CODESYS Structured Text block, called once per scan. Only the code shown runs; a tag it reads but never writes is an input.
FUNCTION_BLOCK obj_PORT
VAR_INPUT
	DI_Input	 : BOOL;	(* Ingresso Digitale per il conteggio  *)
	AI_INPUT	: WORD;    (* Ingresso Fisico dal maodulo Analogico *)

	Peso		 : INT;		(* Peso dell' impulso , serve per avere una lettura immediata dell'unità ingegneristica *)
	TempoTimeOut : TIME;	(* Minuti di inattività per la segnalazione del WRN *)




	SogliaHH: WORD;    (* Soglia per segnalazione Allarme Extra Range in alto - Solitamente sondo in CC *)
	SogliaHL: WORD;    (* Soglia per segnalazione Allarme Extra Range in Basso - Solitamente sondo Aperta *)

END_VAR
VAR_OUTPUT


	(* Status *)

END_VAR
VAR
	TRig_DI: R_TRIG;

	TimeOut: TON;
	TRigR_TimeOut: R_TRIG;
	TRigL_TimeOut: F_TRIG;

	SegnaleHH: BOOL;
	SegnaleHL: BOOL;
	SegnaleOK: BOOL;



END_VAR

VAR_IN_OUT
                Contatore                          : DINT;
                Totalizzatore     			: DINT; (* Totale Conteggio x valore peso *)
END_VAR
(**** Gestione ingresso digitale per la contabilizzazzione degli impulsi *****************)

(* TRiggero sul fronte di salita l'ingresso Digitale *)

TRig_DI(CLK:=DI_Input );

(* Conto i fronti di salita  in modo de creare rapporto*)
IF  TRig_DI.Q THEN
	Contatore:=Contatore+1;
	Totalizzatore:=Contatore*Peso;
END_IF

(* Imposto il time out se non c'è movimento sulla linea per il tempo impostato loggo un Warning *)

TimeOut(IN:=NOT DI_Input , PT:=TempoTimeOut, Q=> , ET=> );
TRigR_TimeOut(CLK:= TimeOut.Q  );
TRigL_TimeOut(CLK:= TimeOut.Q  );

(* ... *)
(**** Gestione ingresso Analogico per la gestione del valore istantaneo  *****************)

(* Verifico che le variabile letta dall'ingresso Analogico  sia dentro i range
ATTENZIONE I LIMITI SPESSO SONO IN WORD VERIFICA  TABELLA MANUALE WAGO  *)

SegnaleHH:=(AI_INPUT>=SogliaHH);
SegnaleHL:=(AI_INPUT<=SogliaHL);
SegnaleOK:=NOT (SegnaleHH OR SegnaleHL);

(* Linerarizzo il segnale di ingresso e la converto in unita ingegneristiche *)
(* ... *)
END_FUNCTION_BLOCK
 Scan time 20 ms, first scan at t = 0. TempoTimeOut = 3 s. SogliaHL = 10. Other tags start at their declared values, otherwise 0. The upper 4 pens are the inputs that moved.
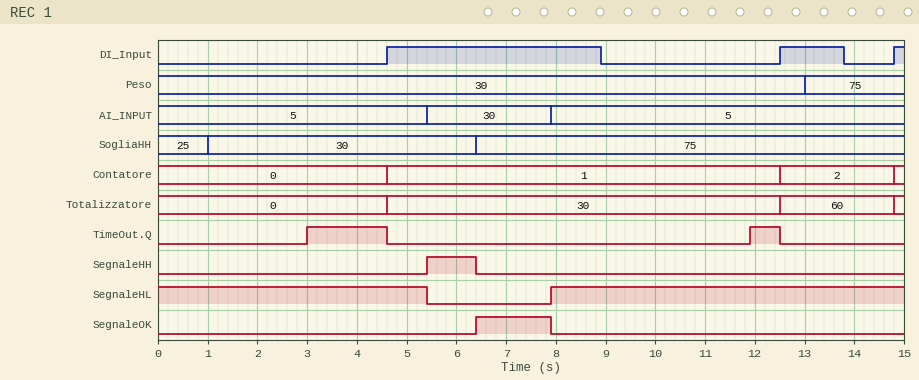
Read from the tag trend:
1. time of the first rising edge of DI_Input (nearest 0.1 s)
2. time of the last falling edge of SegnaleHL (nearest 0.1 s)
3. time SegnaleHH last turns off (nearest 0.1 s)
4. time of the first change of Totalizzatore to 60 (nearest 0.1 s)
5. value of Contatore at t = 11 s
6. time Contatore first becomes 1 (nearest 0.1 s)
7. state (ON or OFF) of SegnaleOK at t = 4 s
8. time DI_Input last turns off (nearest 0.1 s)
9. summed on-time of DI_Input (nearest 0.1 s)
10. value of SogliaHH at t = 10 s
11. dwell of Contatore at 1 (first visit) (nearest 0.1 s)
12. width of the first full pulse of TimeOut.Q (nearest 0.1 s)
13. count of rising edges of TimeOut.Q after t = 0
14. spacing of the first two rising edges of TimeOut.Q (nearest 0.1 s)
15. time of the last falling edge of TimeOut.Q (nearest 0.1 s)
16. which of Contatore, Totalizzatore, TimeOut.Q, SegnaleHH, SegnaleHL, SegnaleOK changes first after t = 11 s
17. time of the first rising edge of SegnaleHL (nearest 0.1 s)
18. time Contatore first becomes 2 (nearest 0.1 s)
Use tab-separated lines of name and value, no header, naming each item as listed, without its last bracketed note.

time of the first rising edge of DI_Input	4.6 s
time of the last falling edge of SegnaleHL	5.4 s
time SegnaleHH last turns off	6.4 s
time of the first change of Totalizzatore to 60	12.5 s
value of Contatore at t = 11 s	1
time Contatore first becomes 1	4.6 s
state (ON or OFF) of SegnaleOK at t = 4 s	OFF
time DI_Input last turns off	13.8 s
summed on-time of DI_Input	5.8 s
value of SogliaHH at t = 10 s	75
dwell of Contatore at 1 (first visit)	7.9 s
width of the first full pulse of TimeOut.Q	1.6 s
count of rising edges of TimeOut.Q after t = 0	2
spacing of the first two rising edges of TimeOut.Q	8.9 s
time of the last falling edge of TimeOut.Q	12.5 s
which of Contatore, Totalizzatore, TimeOut.Q, SegnaleHH, SegnaleHL, SegnaleOK changes first after t = 11 s	TimeOut.Q
time of the first rising edge of SegnaleHL	7.9 s
time Contatore first becomes 2	12.5 s
